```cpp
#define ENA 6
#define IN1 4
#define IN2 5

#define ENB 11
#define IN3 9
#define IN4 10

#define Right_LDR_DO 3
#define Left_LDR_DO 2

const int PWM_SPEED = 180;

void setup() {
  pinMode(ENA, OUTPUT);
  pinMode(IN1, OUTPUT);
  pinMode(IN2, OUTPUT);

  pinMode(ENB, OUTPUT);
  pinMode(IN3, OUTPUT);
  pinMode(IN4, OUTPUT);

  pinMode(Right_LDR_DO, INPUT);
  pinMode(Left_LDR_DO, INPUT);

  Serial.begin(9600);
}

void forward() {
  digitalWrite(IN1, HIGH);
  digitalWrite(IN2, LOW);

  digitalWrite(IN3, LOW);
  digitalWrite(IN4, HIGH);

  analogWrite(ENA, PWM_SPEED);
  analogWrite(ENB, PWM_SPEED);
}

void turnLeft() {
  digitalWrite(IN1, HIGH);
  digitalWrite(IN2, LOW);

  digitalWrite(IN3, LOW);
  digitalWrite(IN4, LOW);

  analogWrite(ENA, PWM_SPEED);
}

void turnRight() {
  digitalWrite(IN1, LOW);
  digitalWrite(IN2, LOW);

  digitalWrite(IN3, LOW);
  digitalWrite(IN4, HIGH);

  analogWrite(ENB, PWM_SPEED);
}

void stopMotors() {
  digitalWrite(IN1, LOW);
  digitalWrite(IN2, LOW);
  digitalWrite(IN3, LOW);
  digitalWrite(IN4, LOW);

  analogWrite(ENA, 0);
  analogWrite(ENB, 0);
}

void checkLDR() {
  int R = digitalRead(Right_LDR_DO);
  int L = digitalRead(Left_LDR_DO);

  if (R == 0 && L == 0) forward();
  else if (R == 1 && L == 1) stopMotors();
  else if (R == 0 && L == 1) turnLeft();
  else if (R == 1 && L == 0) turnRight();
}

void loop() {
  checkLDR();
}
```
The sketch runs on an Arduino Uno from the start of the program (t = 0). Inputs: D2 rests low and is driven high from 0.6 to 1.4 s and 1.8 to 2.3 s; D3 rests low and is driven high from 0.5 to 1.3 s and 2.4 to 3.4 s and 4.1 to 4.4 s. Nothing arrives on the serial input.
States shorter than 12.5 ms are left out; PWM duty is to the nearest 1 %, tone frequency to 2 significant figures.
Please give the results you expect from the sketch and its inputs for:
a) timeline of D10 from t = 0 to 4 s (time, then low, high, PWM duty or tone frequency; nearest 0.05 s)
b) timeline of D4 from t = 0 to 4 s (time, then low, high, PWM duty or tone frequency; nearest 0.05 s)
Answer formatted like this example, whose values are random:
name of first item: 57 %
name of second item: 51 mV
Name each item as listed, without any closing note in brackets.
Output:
timeline of D10 from t = 0 to 4 s: 0 s high; 0.6 s low; 1.4 s high; 1.8 s low; 2.3 s high
timeline of D4 from t = 0 to 4 s: 0 s high; 0.5 s low; 1.3 s high; 2.4 s low; 3.4 s high
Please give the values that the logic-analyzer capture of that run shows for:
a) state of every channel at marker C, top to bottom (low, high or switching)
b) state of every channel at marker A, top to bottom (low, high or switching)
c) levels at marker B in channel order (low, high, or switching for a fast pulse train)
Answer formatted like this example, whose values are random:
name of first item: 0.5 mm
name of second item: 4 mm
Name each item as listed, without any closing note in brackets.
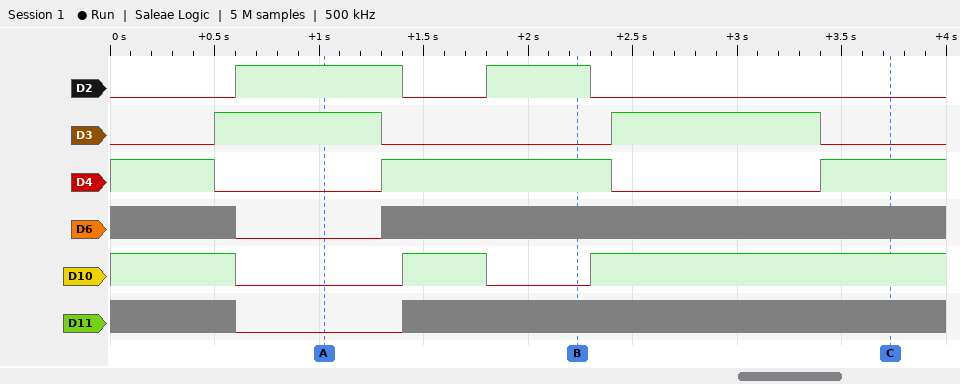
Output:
state of every channel at marker C, top to bottom: D2 low, D3 low, D4 high, D6 switching, D10 high, D11 switching
state of every channel at marker A, top to bottom: D2 high, D3 high, D4 low, D6 low, D10 low, D11 low
levels at marker B in channel order: D2 high, D3 low, D4 high, D6 switching, D10 low, D11 switching
